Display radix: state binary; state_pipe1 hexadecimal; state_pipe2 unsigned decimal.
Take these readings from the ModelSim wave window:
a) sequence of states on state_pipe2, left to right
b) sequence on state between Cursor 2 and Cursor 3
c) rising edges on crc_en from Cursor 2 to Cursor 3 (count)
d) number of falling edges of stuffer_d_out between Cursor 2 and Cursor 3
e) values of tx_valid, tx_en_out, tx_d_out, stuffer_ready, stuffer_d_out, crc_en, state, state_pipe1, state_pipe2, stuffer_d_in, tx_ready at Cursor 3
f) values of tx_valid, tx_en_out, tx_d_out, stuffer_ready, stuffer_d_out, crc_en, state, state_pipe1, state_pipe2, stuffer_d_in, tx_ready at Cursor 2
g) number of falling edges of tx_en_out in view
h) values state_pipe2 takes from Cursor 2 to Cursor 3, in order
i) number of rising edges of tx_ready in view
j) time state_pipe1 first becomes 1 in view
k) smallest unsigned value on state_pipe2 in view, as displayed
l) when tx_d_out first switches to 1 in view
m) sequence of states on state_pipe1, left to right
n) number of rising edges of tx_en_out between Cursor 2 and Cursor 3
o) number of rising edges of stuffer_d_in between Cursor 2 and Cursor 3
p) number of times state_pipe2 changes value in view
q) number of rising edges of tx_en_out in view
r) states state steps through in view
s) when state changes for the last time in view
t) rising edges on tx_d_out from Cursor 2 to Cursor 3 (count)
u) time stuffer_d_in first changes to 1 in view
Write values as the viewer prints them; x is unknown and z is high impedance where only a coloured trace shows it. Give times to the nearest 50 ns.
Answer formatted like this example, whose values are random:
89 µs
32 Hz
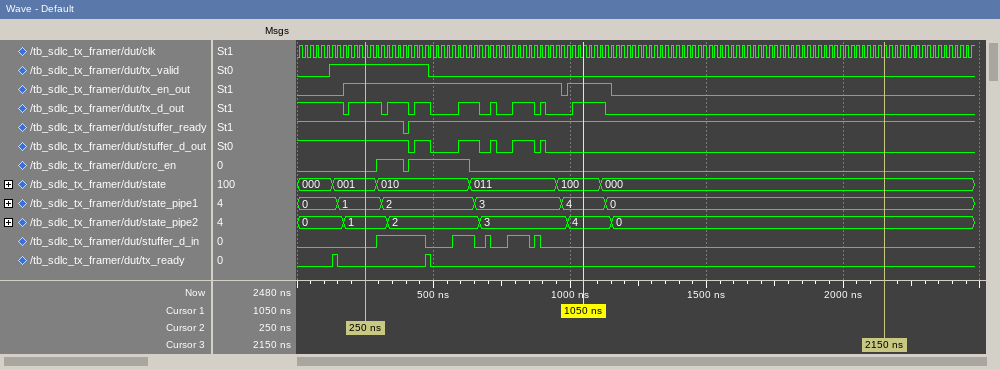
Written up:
0, 1, 2, 3, 4, 0
001, 010, 011, 100, 000
2
6
tx_valid=0, tx_en_out=0, tx_d_out=0, stuffer_ready=1, stuffer_d_out=0, crc_en=0, state=000, state_pipe1=0, state_pipe2=0, stuffer_d_in=0, tx_ready=0
tx_valid=1, tx_en_out=1, tx_d_out=1, stuffer_ready=1, stuffer_d_out=1, crc_en=0, state=001, state_pipe1=1, state_pipe2=1, stuffer_d_in=0, tx_ready=0
2
1, 2, 3, 4, 0
2
150 ns
0
200 ns
0, 1, 2, 3, 4, 0
1
5
5
2
000, 001, 010, 011, 100, 000
1100 ns
7
300 ns
